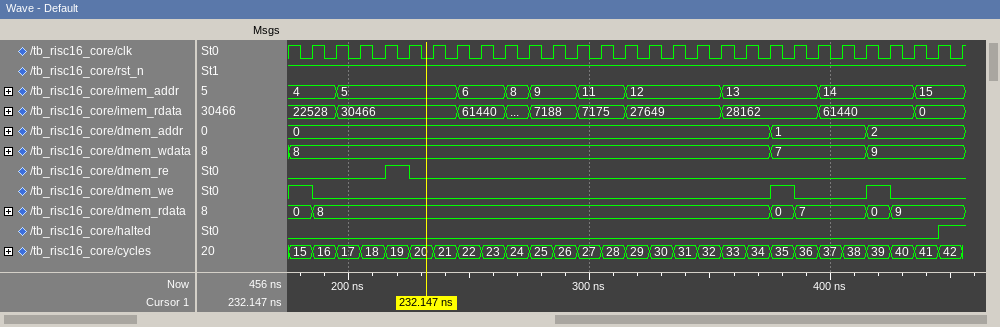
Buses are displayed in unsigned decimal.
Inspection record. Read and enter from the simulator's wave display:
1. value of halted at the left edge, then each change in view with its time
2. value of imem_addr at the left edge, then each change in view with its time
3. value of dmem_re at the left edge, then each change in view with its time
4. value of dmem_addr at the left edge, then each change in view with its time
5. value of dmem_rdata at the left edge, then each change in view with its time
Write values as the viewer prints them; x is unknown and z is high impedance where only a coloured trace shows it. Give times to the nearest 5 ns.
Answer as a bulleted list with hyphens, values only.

- 0, 1 at 445 ns
- 4, 5 at 195 ns, 6 at 245 ns, 8 at 265 ns, 9 at 275 ns, 11 at 295 ns, 12 at 315 ns, 13 at 355 ns, 14 at 395 ns, 15 at 435 ns
- 0, 1 at 215 ns, 0 at 225 ns
- 0, 1 at 375 ns, 2 at 415 ns
- 0, 8 at 185 ns, 0 at 375 ns, 7 at 385 ns, 0 at 415 ns, 9 at 425 ns
